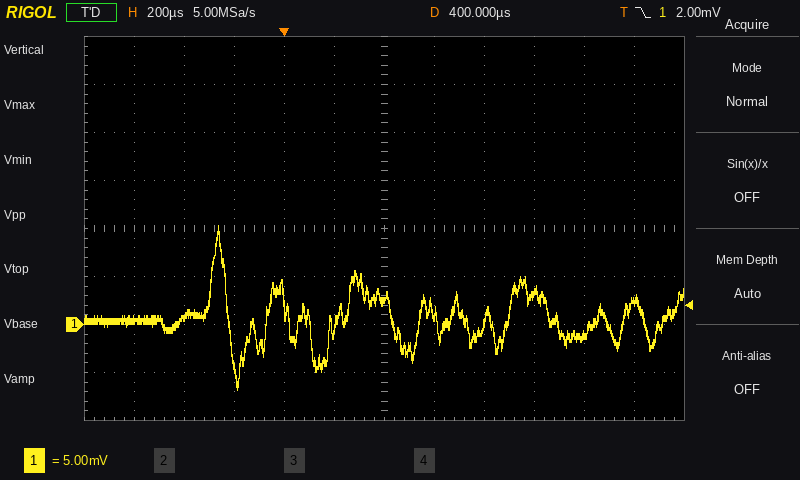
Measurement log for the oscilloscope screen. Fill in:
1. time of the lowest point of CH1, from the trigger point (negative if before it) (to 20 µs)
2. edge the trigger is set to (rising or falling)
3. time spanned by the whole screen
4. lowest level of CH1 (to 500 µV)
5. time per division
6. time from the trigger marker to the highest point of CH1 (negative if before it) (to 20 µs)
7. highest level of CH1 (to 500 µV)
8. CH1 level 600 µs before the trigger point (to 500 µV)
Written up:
-180 µs
falling
2.4 ms
-7.0 mV
200 µs
-260 µs
10.5 mV
500 µV
